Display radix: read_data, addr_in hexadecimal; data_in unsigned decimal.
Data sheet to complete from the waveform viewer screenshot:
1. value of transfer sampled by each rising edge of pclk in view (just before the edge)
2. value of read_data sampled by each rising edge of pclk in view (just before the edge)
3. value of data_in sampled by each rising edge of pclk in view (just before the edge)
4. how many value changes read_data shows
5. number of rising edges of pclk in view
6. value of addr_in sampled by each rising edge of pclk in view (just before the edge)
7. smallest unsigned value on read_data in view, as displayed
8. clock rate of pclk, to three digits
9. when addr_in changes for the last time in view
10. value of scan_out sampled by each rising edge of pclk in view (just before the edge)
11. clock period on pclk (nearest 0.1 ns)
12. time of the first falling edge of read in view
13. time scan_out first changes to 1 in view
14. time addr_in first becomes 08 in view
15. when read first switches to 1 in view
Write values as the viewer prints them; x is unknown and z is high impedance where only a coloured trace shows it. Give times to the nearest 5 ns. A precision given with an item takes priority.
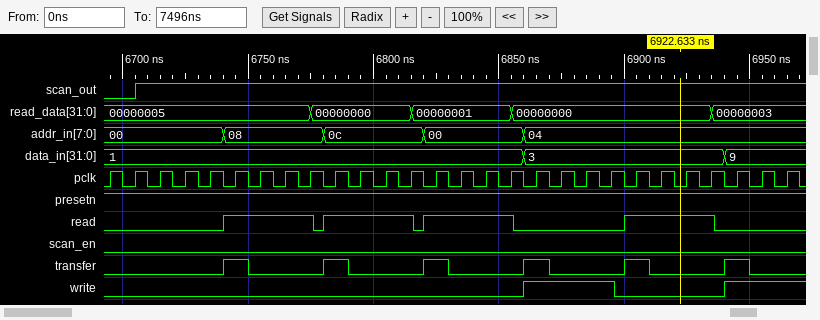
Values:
0 0 0 0 0 1 0 0 0 1 0 0 0 1 0 0 0 1 0 0 0 1 0 0 0 1 0 0
00000005, 00000005, 00000005, 00000005, 00000005, 00000005, 00000005, 00000005, 00000005, 00000000, 00000000, 00000000, 00000000, 00000001, 00000001, 00000001, 00000001, 00000000, 00000000, 00000000, 00000000, 00000000, 00000000, 00000000, 00000000, 00000003, 00000003, 00000003
1, 1, 1, 1, 1, 1, 1, 1, 1, 1, 1, 1, 1, 1, 1, 1, 1, 3, 3, 3, 3, 3, 3, 3, 3, 9, 9, 9
4
28
00, 00, 00, 00, 00, 08, 08, 08, 08, 0c, 0c, 0c, 0c, 00, 00, 00, 00, 04, 04, 04, 04, 04, 04, 04, 04, 04, 04, 04
00000000
100 MHz
6860 ns
0 0 1 1 1 1 1 1 1 1 1 1 1 1 1 1 1 1 1 1 1 1 1 1 1 1 1 1
10 ns
6775 ns
6705 ns
6740 ns
6740 ns
